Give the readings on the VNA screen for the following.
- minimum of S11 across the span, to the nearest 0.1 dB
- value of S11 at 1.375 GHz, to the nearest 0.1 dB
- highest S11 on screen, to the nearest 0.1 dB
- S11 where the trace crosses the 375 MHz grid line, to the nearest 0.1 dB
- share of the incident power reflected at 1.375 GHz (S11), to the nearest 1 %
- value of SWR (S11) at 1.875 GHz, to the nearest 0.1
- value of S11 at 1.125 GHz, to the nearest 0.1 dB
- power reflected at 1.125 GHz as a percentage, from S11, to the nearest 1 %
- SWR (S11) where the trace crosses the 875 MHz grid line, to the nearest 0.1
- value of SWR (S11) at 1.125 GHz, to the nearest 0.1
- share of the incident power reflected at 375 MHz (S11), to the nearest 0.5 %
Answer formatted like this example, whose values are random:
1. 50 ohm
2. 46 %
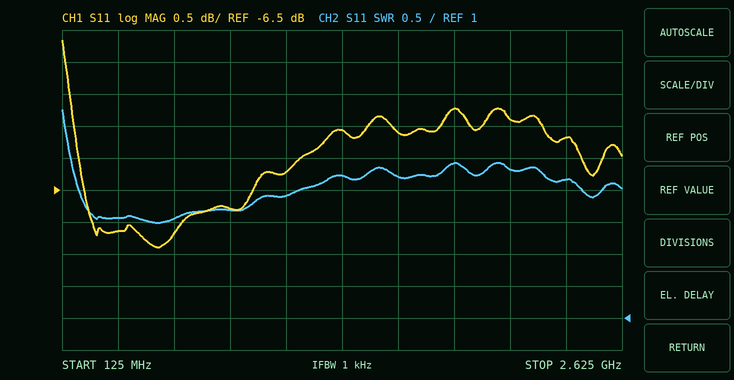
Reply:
1. -7.4 dB
2. -5.6 dB
3. -4.2 dB
4. -7.1 dB
5. 28 %
6. 3.4
7. -6.2 dB
8. 24 %
9. 2.7
10. 2.9
11. 19.5 %
